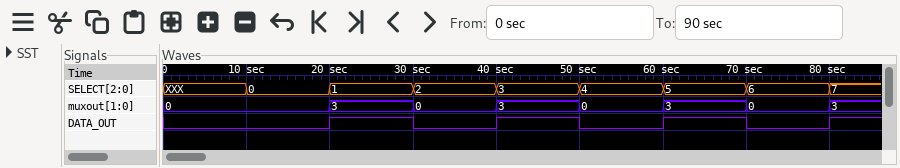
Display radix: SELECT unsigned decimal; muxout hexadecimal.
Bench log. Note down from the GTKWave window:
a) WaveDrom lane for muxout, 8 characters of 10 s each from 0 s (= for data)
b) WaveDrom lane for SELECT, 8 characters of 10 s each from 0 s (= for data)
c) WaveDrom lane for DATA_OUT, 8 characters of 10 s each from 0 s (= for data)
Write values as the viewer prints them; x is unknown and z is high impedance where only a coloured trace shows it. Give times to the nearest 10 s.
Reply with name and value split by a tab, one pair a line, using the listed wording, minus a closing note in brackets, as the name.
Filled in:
WaveDrom lane for muxout, 8 characters of 10 s each from 0 s	{name: 'muxout', wave: '=.======', data: '0 3 0 3 0 3 0'}
WaveDrom lane for SELECT, 8 characters of 10 s each from 0 s	{name: 'SELECT', wave: 'x=======', data: '0 1 2 3 4 5 6'}
WaveDrom lane for DATA_OUT, 8 characters of 10 s each from 0 s	{name: 'DATA_OUT', wave: '0.101010'}
